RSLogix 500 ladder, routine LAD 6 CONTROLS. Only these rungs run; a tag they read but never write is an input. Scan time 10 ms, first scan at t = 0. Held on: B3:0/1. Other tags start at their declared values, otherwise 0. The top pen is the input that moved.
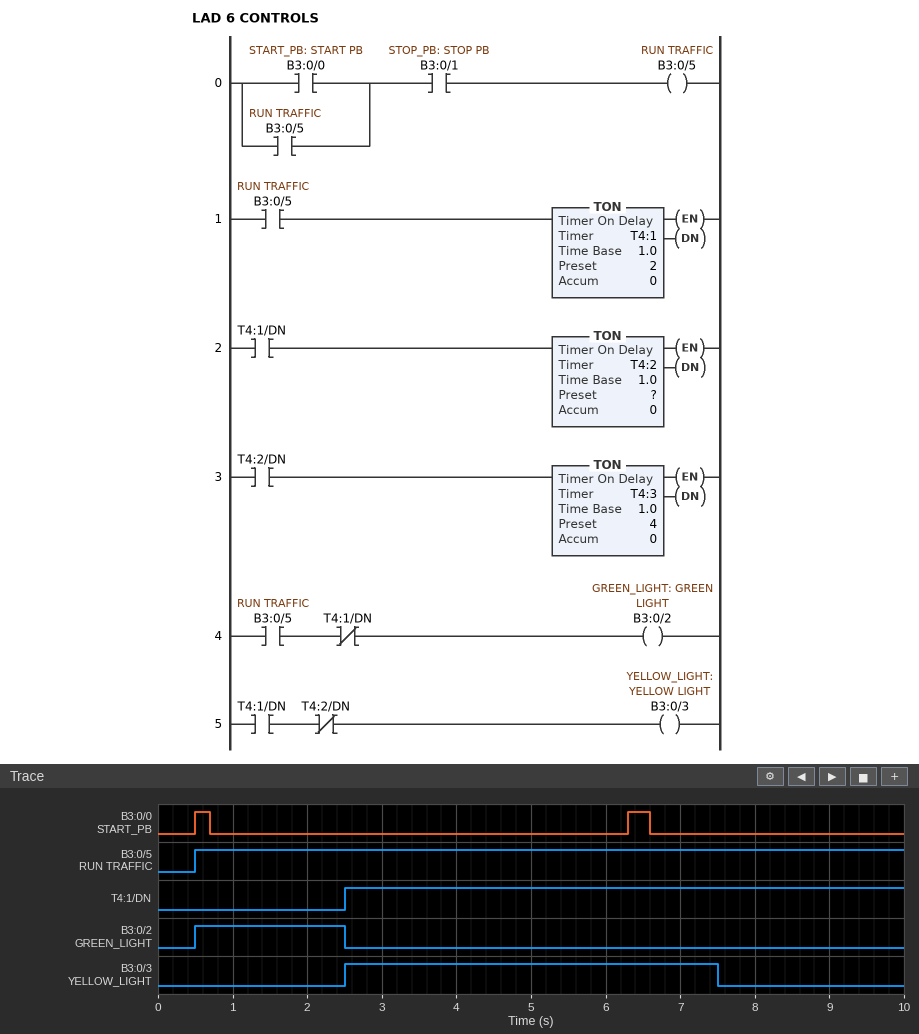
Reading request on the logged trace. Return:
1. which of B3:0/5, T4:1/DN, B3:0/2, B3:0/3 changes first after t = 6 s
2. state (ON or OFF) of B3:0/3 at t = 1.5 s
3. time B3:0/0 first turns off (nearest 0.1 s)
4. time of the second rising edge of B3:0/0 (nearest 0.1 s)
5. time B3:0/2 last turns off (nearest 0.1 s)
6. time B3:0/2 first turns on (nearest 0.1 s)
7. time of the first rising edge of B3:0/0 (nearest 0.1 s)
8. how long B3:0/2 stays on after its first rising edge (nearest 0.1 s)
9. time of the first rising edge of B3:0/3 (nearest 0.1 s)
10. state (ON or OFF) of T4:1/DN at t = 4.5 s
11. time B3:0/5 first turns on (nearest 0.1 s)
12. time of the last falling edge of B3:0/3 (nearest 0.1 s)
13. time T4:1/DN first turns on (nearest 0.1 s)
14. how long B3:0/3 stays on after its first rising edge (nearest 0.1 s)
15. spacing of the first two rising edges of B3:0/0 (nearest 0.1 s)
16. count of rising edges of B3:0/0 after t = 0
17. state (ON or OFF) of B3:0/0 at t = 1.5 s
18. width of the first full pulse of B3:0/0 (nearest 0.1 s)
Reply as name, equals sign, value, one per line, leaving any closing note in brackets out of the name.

which of B3:0/5, T4:1/DN, B3:0/2, B3:0/3 changes first after t = 6 s = B3:0/3
state (ON or OFF) of B3:0/3 at t = 1.5 s = OFF
time B3:0/0 first turns off = 0.7 s
time of the second rising edge of B3:0/0 = 6.3 s
time B3:0/2 last turns off = 2.5 s
time B3:0/2 first turns on = 0.5 s
time of the first rising edge of B3:0/0 = 0.5 s
how long B3:0/2 stays on after its first rising edge = 2.0 s
time of the first rising edge of B3:0/3 = 2.5 s
state (ON or OFF) of T4:1/DN at t = 4.5 s = ON
time B3:0/5 first turns on = 0.5 s
time of the last falling edge of B3:0/3 = 7.5 s
time T4:1/DN first turns on = 2.5 s
how long B3:0/3 stays on after its first rising edge = 5.0 s
spacing of the first two rising edges of B3:0/0 = 5.8 s
count of rising edges of B3:0/0 after t = 0 = 2
state (ON or OFF) of B3:0/0 at t = 1.5 s = OFF
width of the first full pulse of B3:0/0 = 0.2 s
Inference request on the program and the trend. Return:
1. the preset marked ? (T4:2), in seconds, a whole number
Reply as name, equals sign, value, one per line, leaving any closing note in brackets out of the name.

the preset marked ? (T4:2), in seconds, a whole number = 5 s
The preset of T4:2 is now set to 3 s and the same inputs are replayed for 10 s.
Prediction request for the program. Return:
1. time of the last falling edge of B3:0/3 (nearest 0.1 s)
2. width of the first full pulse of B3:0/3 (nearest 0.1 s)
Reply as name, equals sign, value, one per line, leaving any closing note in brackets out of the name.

time of the last falling edge of B3:0/3 = 5.5 s
width of the first full pulse of B3:0/3 = 3.0 s
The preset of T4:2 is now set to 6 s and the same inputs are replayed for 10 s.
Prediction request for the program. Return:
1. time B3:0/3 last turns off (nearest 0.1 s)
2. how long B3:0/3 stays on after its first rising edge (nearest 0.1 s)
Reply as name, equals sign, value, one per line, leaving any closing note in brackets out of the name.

time B3:0/3 last turns off = 8.5 s
how long B3:0/3 stays on after its first rising edge = 6.0 s
